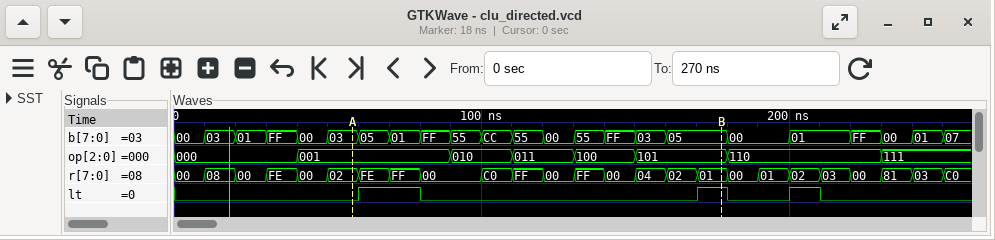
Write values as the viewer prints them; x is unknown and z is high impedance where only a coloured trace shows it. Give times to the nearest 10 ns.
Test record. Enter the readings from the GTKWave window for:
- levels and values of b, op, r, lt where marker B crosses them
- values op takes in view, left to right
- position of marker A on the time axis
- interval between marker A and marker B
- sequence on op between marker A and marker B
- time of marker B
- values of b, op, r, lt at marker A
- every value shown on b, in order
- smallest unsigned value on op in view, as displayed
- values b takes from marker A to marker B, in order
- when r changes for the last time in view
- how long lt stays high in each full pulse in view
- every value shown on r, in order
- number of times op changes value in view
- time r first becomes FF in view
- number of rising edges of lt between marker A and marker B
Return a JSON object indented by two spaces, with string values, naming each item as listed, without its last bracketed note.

{
  "levels and values of b, op, r, lt where marker B crosses them": "b=05, op=101, r=01, lt=1",
  "values op takes in view, left to right": "000, 001, 010, 011, 100, 101, 110, 111",
  "position of marker A on the time axis": "60 ns",
  "interval between marker A and marker B": "120 ns",
  "sequence on op between marker A and marker B": "001, 010, 011, 100, 101",
  "time of marker B": "180 ns",
  "values of b, op, r, lt at marker A": "b=03, op=001, r=02, lt=0",
  "every value shown on b, in order": "00, 03, 01, FF, 00, 03, 05, 01, FF, 55, CC, 55, 00, 55, FF, 03, 05, 00, 01, FF, 00, 01, 07",
  "smallest unsigned value on op in view, as displayed": "000",
  "values b takes from marker A to marker B, in order": "03, 05, 01, FF, 55, CC, 55, 00, 55, FF, 03, 05",
  "when r changes for the last time in view": "250 ns",
  "how long lt stays high in each full pulse in view": "20 ns, 10 ns, 10 ns",
  "every value shown on r, in order": "00, 08, 00, FE, 00, 02, FE, FF, 00, C0, FF, 00, FF, 00, 04, 02, 01, 00, 01, 02, 03, 00, 81, 03, C0",
  "number of times op changes value in view": "7",
  "time r first becomes FF in view": "70 ns",
  "number of rising edges of lt between marker A and marker B": "2"
}
